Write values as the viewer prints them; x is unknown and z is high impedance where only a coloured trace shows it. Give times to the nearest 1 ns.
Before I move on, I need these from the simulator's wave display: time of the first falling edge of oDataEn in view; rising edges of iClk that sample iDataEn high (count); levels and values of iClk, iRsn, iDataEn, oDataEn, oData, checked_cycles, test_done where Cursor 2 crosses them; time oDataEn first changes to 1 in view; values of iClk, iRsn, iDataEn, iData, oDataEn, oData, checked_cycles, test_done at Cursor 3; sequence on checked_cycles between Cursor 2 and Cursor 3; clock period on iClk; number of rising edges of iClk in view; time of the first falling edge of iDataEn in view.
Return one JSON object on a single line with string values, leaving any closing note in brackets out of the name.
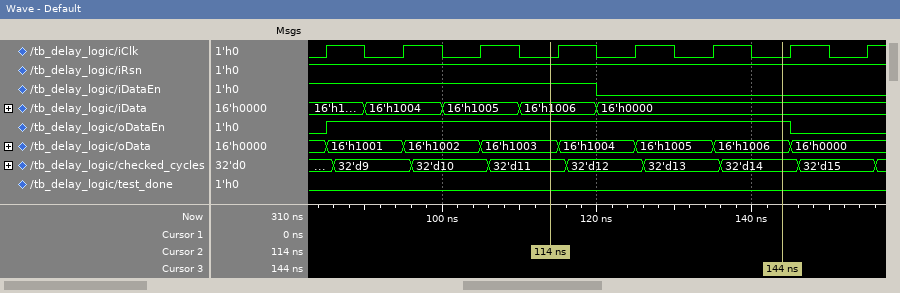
{"time of the first falling edge of oDataEn in view": "145 ns", "rising edges of iClk that sample iDataEn high": "4", "levels and values of iClk, iRsn, iDataEn, oDataEn, oData, checked_cycles, test_done where Cursor 2 crosses them": "iClk=0, iRsn=1, iDataEn=1, oDataEn=1, oData=16'h1003, checked_cycles=32'd11, test_done=0", "time oDataEn first changes to 1 in view": "85 ns", "values of iClk, iRsn, iDataEn, iData, oDataEn, oData, checked_cycles, test_done at Cursor 3": "iClk=0, iRsn=1, iDataEn=0, iData=16'h0000, oDataEn=1, oData=16'h1006, checked_cycles=32'd14, test_done=0", "sequence on checked_cycles between Cursor 2 and Cursor 3": "32'd11, 32'd12, 32'd13, 32'd14", "clock period on iClk": "10 ns", "number of rising edges of iClk in view": "8", "time of the first falling edge of iDataEn in view": "120 ns"}
